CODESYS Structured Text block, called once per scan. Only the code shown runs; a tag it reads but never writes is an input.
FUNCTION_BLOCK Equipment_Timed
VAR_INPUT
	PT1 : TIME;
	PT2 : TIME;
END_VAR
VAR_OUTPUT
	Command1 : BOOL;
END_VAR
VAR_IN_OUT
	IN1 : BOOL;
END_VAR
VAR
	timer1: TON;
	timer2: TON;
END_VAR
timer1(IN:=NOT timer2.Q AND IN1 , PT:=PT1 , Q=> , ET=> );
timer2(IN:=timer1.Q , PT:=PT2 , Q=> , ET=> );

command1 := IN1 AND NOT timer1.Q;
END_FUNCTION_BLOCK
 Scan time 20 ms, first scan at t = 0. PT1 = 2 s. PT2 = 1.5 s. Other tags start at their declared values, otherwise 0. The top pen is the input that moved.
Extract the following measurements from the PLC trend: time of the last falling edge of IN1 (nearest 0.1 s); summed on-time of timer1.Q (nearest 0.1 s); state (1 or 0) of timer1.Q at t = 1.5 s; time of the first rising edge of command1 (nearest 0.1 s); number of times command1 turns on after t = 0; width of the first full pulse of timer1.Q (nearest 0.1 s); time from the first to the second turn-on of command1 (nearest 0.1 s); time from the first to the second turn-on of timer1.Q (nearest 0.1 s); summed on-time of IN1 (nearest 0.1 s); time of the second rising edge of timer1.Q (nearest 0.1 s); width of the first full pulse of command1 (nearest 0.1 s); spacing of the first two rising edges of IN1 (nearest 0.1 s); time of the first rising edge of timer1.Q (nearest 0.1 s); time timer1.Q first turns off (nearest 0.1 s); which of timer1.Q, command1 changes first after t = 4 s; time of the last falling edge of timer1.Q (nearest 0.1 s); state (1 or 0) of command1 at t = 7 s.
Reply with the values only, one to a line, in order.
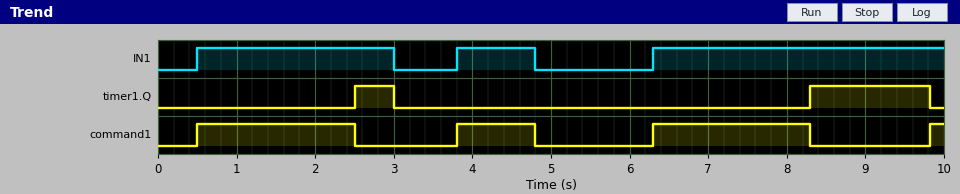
4.8 s
2.0 s
0
0.5 s
4
0.5 s
3.3 s
5.8 s
7.2 s
8.3 s
2.0 s
3.3 s
2.5 s
3.0 s
command1
9.8 s
1
